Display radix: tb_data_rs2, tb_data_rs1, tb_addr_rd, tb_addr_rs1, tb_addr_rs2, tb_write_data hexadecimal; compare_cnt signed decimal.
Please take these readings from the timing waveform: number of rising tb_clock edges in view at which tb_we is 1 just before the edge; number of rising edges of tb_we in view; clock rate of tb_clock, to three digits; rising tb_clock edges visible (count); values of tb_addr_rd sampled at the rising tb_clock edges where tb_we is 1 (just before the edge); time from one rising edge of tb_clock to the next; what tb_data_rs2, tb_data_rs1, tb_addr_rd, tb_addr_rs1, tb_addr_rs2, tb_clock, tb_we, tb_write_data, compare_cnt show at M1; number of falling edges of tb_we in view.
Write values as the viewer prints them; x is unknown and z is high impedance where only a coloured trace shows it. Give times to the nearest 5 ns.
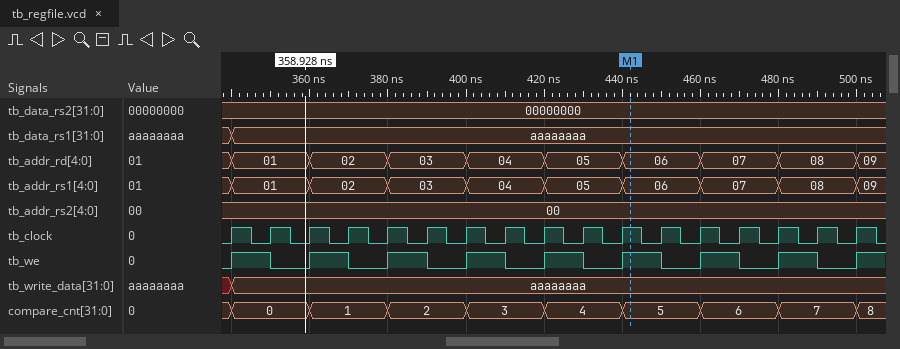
8
9
100 MHz
17
01, 02, 03, 04, 05, 06, 07, 08
10 ns
tb_data_rs2=00000000, tb_data_rs1=aaaaaaaa, tb_addr_rd=06, tb_addr_rs1=06, tb_addr_rs2=00, tb_clock=1, tb_we=1, tb_write_data=aaaaaaaa, compare_cnt=5
8
